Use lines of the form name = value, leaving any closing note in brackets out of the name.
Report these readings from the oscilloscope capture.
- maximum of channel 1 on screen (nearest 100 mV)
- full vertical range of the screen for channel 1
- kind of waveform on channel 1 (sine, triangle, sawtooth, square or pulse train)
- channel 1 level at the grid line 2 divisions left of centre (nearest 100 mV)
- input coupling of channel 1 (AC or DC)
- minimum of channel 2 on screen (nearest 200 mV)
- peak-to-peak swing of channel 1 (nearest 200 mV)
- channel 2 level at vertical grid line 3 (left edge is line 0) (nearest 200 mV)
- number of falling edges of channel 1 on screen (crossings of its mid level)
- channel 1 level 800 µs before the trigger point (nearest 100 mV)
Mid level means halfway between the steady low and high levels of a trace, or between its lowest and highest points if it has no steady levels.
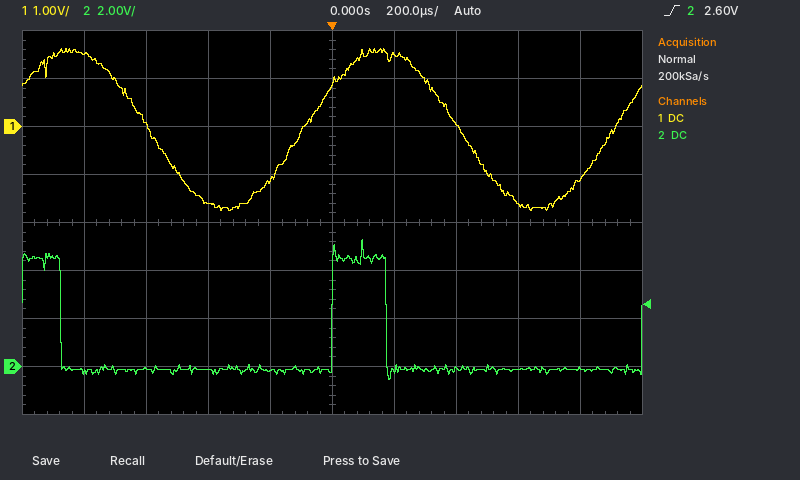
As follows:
maximum of channel 1 on screen = 1.6 V
full vertical range of the screen for channel 1 = 8 V
kind of waveform on channel 1 = sine
channel 1 level at the grid line 2 divisions left of centre = -1.6 V
input coupling of channel 1 = DC
minimum of channel 2 on screen = -600 mV
peak-to-peak swing of channel 1 = 3.4 V
channel 2 level at vertical grid line 3 (left edge is line 0) = -200 mV
number of falling edges of channel 1 on screen = 2
channel 1 level 800 µs before the trigger point = 1.5 V
